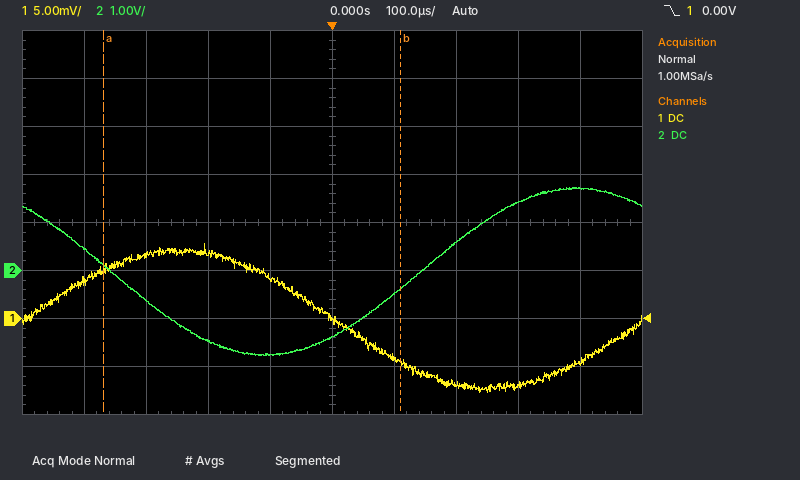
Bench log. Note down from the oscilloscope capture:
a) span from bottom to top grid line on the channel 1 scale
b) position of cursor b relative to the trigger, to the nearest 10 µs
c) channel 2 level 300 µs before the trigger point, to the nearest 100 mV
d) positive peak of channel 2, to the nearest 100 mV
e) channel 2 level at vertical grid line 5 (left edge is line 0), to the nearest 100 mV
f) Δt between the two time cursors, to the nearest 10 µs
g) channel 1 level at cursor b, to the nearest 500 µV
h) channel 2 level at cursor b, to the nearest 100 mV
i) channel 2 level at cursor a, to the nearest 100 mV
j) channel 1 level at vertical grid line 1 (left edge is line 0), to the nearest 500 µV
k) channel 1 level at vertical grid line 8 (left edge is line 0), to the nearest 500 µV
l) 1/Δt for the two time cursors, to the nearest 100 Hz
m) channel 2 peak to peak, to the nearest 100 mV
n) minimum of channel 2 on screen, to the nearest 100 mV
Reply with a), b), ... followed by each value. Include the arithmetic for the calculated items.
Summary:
a) 40 mV
b) +110 µs
c) -600 mV
d) 1.7 V
e) -1.4 V
f) 480 µs
g) -4.5 mV
h) -400 mV
i) 100 mV
j) 4.0 mV
k) -7.0 mV
l) 1 / 480 µs ≈ 2.1 kHz
m) 1.7 V − (-1.8 V) = 3.5 V
n) -1.8 V
